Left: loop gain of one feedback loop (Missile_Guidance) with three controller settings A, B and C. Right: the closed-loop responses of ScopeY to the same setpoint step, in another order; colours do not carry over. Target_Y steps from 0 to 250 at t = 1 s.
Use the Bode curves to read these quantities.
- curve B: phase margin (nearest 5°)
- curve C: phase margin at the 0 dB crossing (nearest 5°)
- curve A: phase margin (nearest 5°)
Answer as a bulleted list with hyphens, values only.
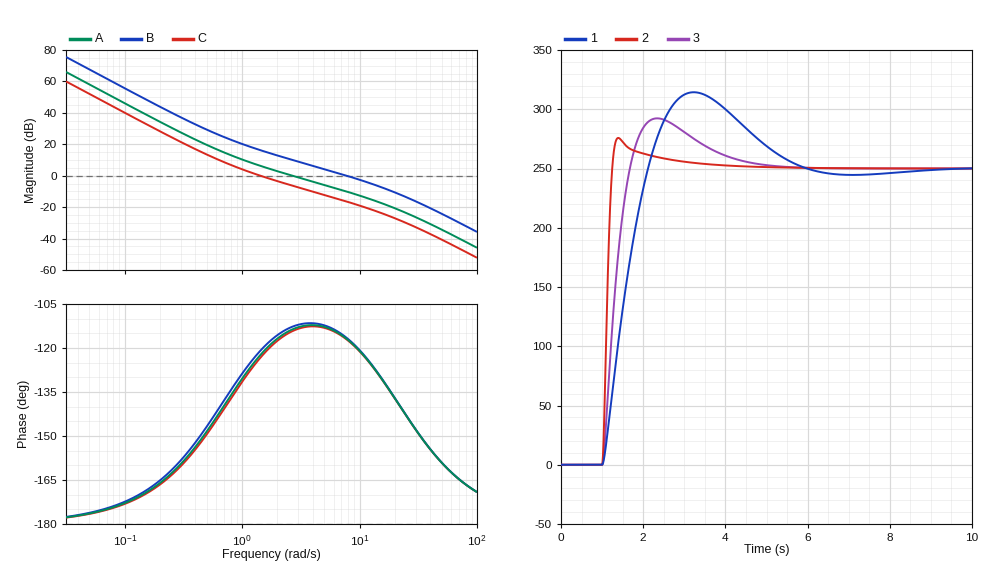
- 65°
- 55°
- 65°
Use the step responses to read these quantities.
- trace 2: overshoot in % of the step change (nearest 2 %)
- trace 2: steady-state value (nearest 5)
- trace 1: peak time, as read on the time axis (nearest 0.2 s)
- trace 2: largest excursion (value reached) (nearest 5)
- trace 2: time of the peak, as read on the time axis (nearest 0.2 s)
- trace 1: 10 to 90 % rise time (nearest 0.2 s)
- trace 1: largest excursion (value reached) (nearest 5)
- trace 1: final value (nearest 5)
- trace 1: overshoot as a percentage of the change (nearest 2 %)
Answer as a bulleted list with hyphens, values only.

- 10 %
- 250
- 3.2 s
- 275
- 1.4 s
- 0.8 s
- 315
- 250
- 26 %
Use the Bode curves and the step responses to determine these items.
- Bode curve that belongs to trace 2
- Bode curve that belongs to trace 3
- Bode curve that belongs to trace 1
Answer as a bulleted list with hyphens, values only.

- B
- A
- C
